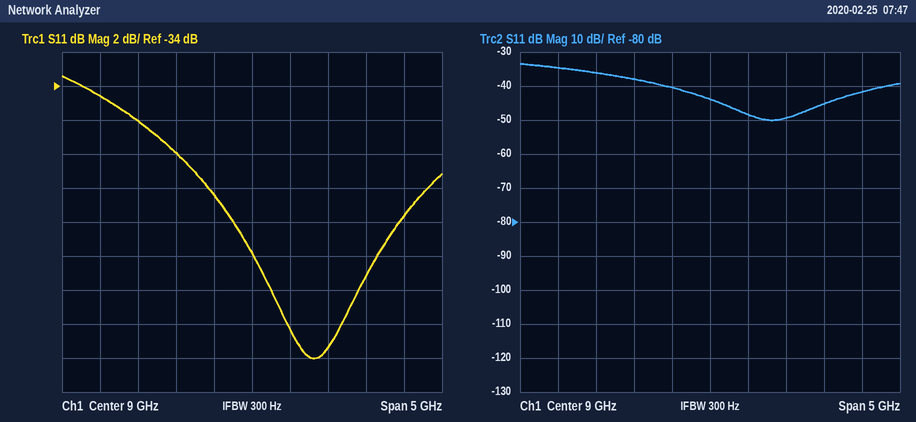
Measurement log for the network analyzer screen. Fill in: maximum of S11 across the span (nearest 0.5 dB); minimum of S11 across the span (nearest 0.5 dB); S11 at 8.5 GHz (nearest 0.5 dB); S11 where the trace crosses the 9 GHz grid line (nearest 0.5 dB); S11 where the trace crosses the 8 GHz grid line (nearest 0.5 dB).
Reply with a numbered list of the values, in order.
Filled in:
1. -33.5 dB
2. -50.0 dB
3. -40.5 dB
4. -44.0 dB
5. -38.0 dB
